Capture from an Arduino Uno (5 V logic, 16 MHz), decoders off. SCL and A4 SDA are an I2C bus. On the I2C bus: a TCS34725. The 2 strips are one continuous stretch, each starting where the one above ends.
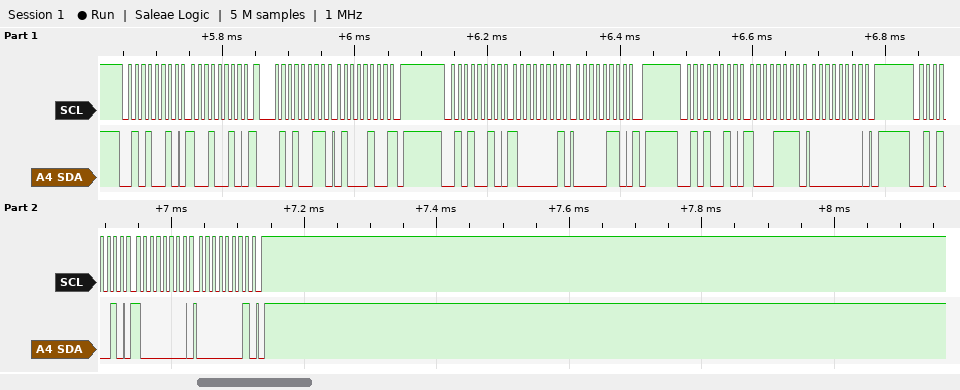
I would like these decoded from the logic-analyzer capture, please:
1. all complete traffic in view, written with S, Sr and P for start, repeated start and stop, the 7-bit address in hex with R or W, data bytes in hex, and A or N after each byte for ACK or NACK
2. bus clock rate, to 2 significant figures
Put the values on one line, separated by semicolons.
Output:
S 29W A 92 A Sr 29R A 44 N P S 29W A 81 A 06 A P S 29W A 8F A 00 A P S 29W A 80 A 01 A P; 100 kHz
